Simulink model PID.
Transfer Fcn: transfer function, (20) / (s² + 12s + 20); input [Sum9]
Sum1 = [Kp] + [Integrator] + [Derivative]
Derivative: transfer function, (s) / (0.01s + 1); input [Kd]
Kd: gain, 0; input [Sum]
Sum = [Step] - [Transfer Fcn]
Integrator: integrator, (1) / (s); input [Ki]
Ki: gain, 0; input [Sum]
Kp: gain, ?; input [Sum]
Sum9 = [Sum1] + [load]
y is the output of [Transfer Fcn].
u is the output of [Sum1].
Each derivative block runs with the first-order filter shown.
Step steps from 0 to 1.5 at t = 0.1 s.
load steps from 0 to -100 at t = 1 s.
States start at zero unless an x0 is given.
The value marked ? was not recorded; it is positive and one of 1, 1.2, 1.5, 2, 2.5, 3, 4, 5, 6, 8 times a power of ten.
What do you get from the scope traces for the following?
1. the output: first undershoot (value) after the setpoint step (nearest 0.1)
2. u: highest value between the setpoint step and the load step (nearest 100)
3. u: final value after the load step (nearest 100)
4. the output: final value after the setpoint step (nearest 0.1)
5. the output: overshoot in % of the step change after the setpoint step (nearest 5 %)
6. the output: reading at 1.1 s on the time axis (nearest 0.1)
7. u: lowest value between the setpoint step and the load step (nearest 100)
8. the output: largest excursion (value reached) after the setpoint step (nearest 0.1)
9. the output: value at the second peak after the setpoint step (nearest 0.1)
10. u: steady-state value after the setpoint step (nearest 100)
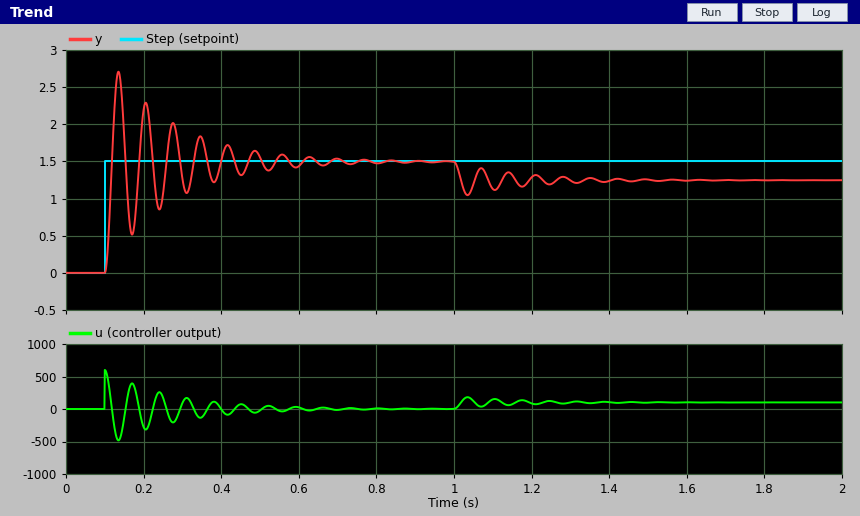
0.5
600
100
1.5
80 %
1.1
-500
2.7
2.3
0
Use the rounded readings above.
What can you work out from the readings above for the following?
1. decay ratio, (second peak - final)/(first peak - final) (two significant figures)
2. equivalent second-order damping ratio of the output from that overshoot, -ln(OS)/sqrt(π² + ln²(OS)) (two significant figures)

0.67
0.071
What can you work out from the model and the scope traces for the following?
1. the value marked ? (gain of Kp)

400
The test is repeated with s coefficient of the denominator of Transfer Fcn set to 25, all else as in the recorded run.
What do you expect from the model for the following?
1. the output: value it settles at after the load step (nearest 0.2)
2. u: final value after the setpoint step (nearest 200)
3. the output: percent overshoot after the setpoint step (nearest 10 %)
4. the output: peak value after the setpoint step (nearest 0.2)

1.2
0
60 %
2.4
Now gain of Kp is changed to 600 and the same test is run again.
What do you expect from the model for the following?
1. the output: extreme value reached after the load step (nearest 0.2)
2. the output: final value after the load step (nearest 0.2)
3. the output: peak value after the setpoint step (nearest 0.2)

1.2
1.4
2.8
